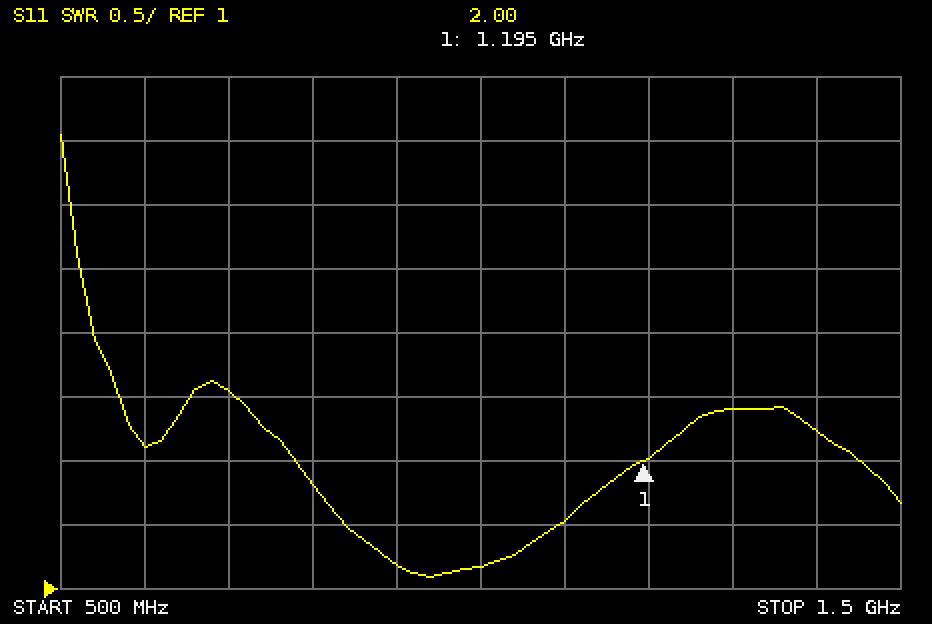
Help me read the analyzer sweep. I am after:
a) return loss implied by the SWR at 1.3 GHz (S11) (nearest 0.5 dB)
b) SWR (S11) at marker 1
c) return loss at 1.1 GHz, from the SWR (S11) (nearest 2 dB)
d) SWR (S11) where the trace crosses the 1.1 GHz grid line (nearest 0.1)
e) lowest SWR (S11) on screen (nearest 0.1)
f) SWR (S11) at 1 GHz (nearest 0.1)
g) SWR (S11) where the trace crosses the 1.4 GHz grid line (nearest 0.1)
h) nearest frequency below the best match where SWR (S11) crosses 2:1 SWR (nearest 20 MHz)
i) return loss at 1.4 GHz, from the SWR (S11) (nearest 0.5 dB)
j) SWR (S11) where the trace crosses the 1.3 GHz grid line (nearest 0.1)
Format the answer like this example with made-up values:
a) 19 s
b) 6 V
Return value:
a) 7.5 dB
b) 2.00
c) 14 dB
d) 1.5
e) 1.1
f) 1.2
g) 2.2
h) 780 MHz
i) 8.5 dB
j) 2.4
